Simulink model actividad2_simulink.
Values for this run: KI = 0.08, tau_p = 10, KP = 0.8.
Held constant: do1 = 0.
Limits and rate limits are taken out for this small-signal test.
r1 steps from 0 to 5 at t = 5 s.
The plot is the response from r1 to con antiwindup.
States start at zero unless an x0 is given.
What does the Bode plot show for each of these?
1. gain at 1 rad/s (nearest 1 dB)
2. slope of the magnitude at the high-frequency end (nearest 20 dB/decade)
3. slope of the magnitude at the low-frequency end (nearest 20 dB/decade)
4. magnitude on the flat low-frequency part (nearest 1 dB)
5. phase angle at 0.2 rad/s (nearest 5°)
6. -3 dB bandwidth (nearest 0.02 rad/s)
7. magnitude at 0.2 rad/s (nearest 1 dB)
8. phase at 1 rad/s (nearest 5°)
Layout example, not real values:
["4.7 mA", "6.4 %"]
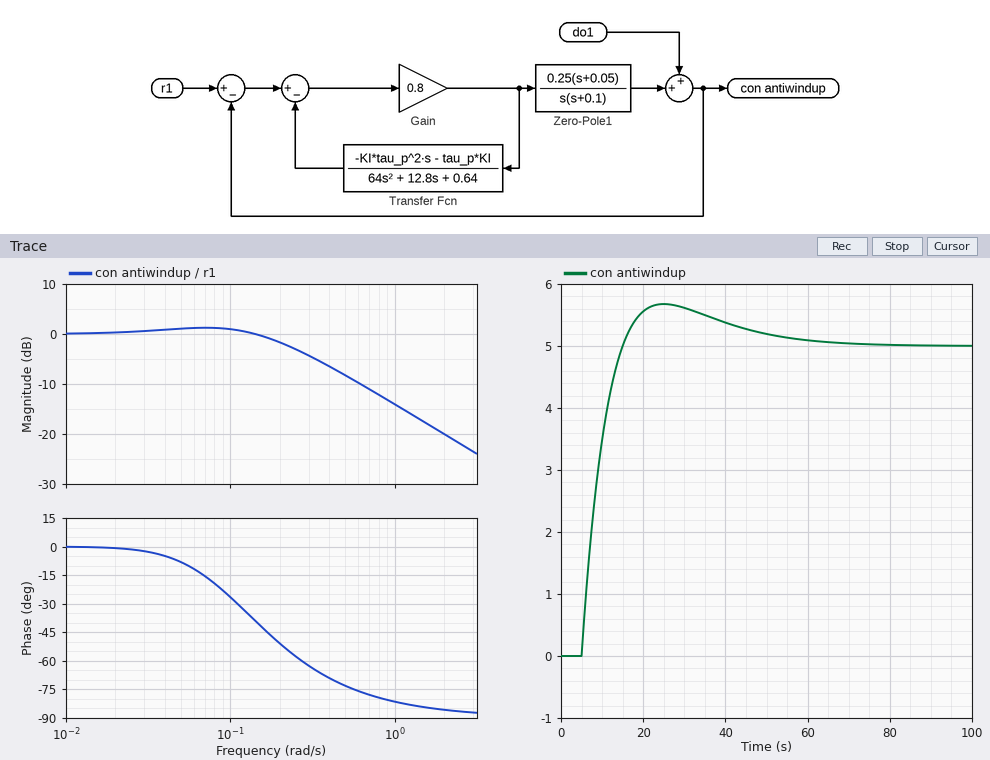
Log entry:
["-14 dB", "-20 dB/decade", "0 dB/decade", "0 dB", "-50°", "0.24 rad/s", "-2 dB", "-80°"]
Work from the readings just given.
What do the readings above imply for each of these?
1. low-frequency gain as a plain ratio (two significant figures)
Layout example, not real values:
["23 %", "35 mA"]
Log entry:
["1.0"]
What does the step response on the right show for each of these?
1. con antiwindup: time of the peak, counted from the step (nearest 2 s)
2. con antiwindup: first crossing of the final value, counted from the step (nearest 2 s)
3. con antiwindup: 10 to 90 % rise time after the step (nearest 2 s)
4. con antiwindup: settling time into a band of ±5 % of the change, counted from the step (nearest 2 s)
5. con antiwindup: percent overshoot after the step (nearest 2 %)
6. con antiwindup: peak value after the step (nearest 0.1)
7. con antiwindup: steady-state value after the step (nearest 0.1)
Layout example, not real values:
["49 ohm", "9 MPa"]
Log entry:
["20 s", "10 s", "8 s", "42 s", "14 %", "5.7", "5.0"]
